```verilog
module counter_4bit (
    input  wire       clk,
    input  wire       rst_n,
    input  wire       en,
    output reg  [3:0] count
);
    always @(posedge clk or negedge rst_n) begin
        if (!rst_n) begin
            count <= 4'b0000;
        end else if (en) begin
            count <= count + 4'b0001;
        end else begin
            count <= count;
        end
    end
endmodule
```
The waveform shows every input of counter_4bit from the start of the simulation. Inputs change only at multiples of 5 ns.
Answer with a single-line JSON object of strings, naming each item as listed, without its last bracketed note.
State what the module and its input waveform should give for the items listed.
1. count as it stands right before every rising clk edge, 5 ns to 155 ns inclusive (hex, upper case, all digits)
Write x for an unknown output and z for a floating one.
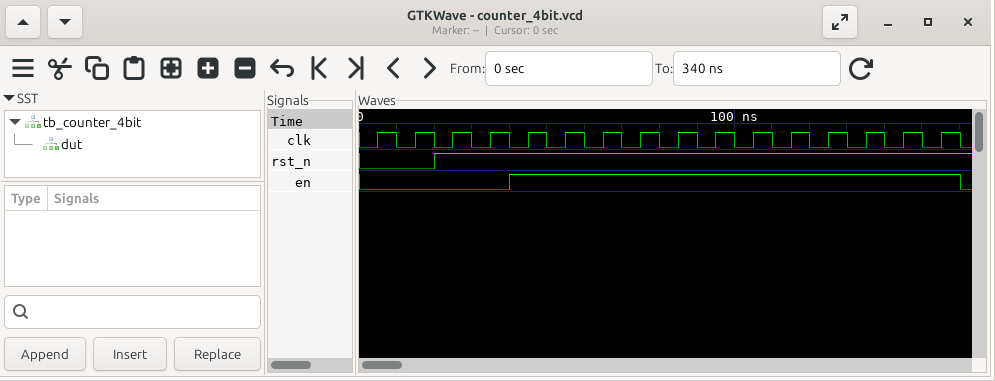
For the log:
{"count as it stands right before every rising clk edge, 5 ns to 155 ns inclusive": "0, 0, 0, 0, 0, 1, 2, 3, 4, 5, 6, 7, 8, 9, A, B"}
